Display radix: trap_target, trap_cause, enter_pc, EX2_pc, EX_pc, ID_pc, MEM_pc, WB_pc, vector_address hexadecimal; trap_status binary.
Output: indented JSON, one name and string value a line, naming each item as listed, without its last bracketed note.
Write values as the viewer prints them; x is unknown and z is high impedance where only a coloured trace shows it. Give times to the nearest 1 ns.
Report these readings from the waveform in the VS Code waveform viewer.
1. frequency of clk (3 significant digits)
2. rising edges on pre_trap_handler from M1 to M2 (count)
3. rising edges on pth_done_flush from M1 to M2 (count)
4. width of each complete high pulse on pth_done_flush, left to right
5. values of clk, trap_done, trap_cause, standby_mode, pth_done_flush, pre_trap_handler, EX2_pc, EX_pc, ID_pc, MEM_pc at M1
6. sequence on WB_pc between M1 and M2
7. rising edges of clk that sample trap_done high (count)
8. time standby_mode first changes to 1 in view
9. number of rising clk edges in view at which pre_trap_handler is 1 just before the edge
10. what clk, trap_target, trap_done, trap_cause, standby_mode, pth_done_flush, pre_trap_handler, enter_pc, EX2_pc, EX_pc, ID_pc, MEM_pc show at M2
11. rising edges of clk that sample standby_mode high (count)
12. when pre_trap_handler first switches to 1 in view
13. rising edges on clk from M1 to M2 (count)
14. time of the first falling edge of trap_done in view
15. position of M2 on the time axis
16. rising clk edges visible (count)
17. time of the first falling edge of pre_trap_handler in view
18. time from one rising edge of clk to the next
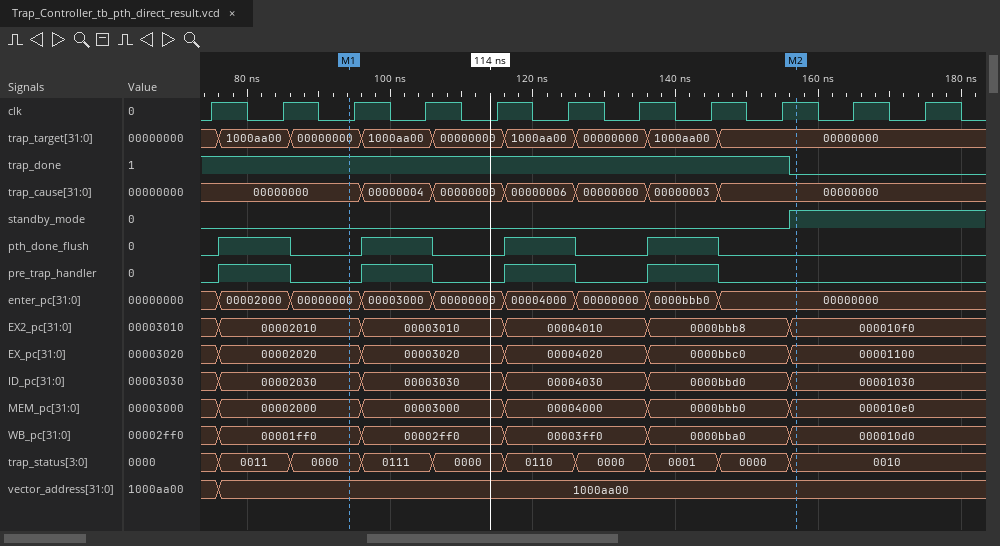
{
  "frequency of clk": "100 MHz",
  "rising edges on pre_trap_handler from M1 to M2": "3",
  "rising edges on pth_done_flush from M1 to M2": "3",
  "width of each complete high pulse on pth_done_flush, left to right": "10 ns, 10 ns, 10 ns, 10 ns",
  "values of clk, trap_done, trap_cause, standby_mode, pth_done_flush, pre_trap_handler, EX2_pc, EX_pc, ID_pc, MEM_pc at M1": "clk=0, trap_done=1, trap_cause=00000000, standby_mode=0, pth_done_flush=0, pre_trap_handler=0, EX2_pc=00002010, EX_pc=00002020, ID_pc=00002030, MEM_pc=00002000",
  "sequence on WB_pc between M1 and M2": "00001ff0, 00002ff0, 00003ff0, 0000bba0, 000010d0",
  "rising edges of clk that sample trap_done high": "9",
  "time standby_mode first changes to 1 in view": "156 ns",
  "number of rising clk edges in view at which pre_trap_handler is 1 just before the edge": "4",
  "what clk, trap_target, trap_done, trap_cause, standby_mode, pth_done_flush, pre_trap_handler, enter_pc, EX2_pc, EX_pc, ID_pc, MEM_pc show at M2": "clk=1, trap_target=00000000, trap_done=0, trap_cause=00000000, standby_mode=1, pth_done_flush=0, pre_trap_handler=0, enter_pc=00000000, EX2_pc=000010f0, EX_pc=00001100, ID_pc=00001030, MEM_pc=000010e0",
  "rising edges of clk that sample standby_mode high": "2",
  "when pre_trap_handler first switches to 1 in view": "76 ns",
  "rising edges on clk from M1 to M2": "7",
  "time of the first falling edge of trap_done in view": "156 ns",
  "position of M2 on the time axis": "157 ns",
  "rising clk edges visible": "11",
  "time of the first falling edge of pre_trap_handler in view": "86 ns",
  "time from one rising edge of clk to the next": "10 ns"
}
